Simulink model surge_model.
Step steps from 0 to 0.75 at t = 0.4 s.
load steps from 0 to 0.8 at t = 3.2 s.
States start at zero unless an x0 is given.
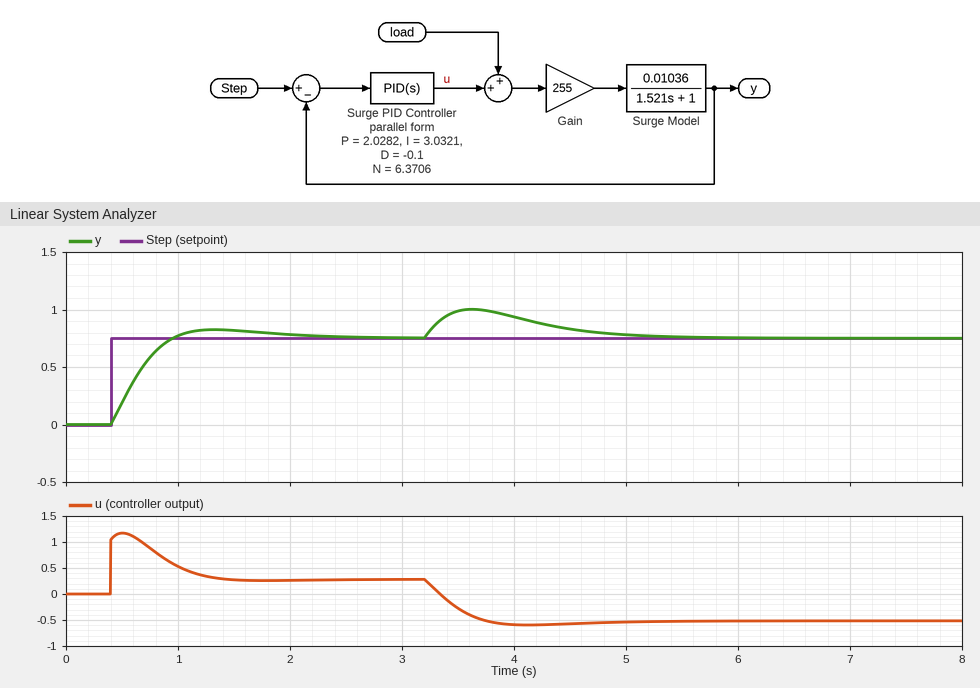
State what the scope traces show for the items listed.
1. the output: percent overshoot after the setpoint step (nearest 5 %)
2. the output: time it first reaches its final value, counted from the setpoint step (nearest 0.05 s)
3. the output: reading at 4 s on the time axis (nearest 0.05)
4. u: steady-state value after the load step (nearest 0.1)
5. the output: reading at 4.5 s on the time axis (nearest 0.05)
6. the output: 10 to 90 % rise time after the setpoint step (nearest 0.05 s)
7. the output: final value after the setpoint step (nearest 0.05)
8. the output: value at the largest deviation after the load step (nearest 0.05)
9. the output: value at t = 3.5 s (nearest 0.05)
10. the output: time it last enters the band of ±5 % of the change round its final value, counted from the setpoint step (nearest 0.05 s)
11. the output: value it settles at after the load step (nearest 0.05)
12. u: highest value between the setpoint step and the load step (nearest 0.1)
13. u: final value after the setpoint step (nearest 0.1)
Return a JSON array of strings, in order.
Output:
["10 %", "0.55 s", "0.95", "-0.5", "0.85", "0.40 s", "0.75", "1.00", "1.00", "1.50 s", "0.75", "1.2", "0.3"]
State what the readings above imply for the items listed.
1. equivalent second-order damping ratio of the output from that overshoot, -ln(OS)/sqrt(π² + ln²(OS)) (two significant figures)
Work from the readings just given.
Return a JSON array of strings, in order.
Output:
["0.59"]
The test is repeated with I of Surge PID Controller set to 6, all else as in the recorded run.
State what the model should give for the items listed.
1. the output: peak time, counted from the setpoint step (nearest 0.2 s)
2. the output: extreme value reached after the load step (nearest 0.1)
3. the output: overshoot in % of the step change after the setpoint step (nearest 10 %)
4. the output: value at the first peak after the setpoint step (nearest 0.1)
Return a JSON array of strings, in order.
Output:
["0.8 s", "1.0", "20 %", "0.9"]
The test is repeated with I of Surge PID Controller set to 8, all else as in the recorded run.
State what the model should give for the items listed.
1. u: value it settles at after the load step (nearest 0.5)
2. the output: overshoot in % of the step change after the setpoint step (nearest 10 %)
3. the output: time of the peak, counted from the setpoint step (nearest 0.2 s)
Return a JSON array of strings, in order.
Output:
["-0.5", "30 %", "0.6 s"]
